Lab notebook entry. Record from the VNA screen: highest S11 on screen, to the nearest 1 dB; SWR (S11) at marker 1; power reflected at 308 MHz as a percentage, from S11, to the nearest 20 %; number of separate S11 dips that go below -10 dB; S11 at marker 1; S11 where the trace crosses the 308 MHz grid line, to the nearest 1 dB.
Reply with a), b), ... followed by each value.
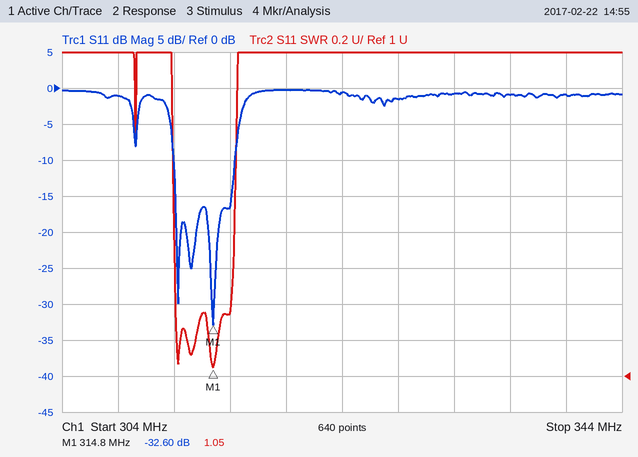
a) 0 dB
b) 1.05
c) 80 %
d) 3
e) -32.60 dB
f) -1 dB
